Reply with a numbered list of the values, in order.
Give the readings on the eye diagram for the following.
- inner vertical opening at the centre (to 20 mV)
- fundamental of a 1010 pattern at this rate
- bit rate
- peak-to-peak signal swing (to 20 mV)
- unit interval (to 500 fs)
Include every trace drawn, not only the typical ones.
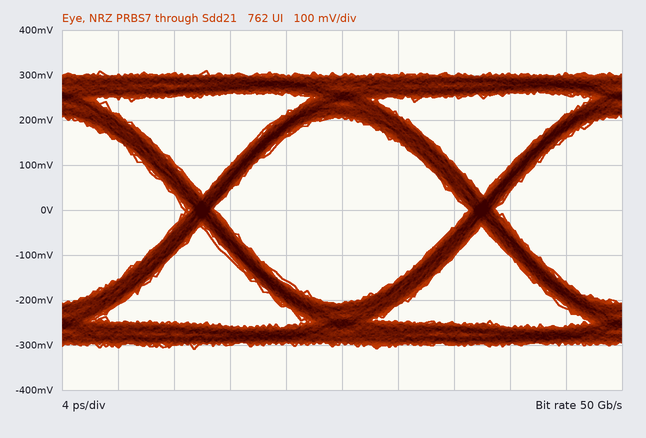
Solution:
1. 420 mV
2. 25 GHz
3. 50 Gb/s
4. 620 mV
5. 20.0 ps
